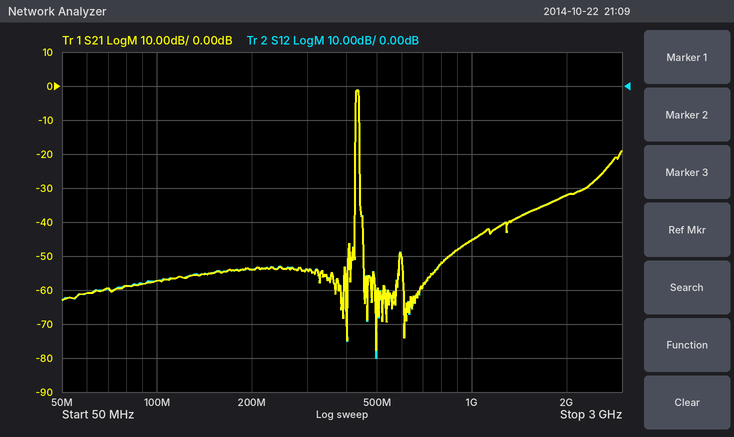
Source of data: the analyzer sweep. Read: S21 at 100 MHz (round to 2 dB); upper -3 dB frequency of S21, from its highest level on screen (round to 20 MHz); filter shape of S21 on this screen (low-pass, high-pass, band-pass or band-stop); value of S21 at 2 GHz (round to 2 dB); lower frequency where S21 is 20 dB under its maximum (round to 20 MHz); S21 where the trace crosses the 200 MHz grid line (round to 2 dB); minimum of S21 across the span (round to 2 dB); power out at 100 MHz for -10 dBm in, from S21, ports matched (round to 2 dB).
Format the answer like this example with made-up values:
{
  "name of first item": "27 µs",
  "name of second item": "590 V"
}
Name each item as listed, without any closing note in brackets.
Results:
{
  "S21 at 100 MHz": "-58 dB",
  "upper -3 dB frequency of S21, from its highest level on screen": "440 MHz",
  "filter shape of S21 on this screen": "band-pass",
  "value of S21 at 2 GHz": "-32 dB",
  "lower frequency where S21 is 20 dB under its maximum": "420 MHz",
  "S21 where the trace crosses the 200 MHz grid line": "-54 dB",
  "minimum of S21 across the span": "-78 dB",
  "power out at 100 MHz for -10 dBm in, from S21, ports matched": "-68 dBm"
}
